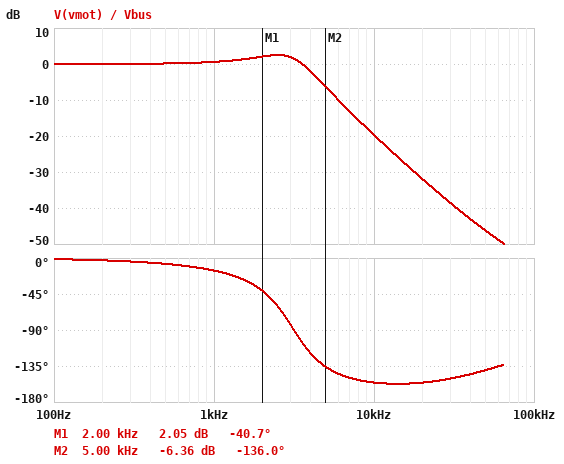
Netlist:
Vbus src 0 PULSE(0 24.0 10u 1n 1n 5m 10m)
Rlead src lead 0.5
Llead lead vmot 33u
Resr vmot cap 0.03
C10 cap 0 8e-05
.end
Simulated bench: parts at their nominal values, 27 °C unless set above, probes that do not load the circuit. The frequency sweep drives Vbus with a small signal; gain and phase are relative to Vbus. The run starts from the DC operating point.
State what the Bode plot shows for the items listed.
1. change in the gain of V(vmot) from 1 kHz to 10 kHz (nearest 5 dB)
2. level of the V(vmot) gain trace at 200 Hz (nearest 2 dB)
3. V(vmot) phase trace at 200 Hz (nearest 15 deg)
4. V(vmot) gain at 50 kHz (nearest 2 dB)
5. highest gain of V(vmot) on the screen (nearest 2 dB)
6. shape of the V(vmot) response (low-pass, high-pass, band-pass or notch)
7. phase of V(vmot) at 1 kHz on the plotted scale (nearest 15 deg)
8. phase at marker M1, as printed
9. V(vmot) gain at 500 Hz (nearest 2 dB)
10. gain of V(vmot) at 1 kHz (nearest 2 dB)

-20 dB
0 dB
0 deg
-46 dB
2 dB
low-pass
-15 deg
-40.7 deg
0 dB
0 dB
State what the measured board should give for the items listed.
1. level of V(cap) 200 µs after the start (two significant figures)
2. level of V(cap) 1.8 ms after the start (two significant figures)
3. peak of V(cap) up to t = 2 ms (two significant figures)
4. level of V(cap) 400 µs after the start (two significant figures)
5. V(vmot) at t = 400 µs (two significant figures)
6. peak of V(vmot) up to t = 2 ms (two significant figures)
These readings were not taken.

30 V
24 V
30 V
23 V
23 V
30 V
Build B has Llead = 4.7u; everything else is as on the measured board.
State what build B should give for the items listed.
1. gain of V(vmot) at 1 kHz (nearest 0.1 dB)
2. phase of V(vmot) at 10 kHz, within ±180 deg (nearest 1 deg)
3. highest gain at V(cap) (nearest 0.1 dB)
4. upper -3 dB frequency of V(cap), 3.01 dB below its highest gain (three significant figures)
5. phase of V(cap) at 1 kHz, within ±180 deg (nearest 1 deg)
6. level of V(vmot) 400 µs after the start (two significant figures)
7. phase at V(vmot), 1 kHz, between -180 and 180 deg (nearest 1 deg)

-0.2 dB
-92 deg
0 dB
4.66 kHz
-15 deg
24 V
-14 deg
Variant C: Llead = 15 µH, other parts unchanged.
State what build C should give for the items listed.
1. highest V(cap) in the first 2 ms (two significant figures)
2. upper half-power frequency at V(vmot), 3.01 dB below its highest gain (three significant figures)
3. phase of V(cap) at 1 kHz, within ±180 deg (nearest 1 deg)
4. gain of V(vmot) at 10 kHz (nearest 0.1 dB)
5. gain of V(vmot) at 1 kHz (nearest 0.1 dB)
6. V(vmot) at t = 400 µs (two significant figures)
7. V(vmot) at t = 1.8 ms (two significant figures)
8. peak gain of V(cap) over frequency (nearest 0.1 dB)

26 V
5.08 kHz
-16 deg
-13.1 dB
0.1 dB
24 V
24 V
0.3 dB
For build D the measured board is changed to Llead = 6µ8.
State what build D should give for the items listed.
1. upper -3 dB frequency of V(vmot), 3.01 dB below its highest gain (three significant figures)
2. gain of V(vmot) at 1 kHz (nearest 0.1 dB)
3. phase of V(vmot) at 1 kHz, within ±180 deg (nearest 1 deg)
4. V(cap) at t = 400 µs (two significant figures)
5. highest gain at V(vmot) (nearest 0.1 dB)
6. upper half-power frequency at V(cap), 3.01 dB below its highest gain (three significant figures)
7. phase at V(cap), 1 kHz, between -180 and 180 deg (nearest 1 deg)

5.04 kHz
-0.1 dB
-14 deg
24 V
0 dB
5.02 kHz
-15 deg
